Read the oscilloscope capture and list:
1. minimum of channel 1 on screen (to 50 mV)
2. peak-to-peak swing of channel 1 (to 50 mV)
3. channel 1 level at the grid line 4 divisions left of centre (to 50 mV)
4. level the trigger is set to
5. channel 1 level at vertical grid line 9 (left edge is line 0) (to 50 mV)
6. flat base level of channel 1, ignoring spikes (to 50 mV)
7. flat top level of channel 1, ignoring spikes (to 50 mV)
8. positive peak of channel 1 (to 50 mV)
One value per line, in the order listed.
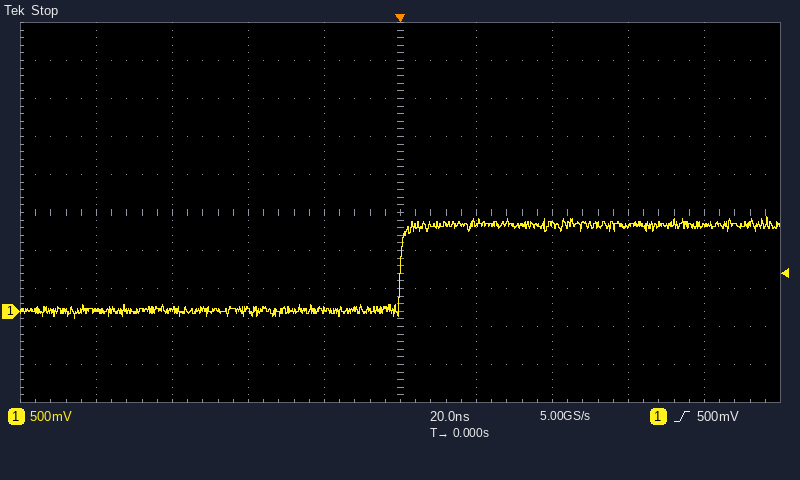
-100 mV
1.35 V
0 mV
500 mV
1.10 V
0 mV
1.15 V
1.25 V
